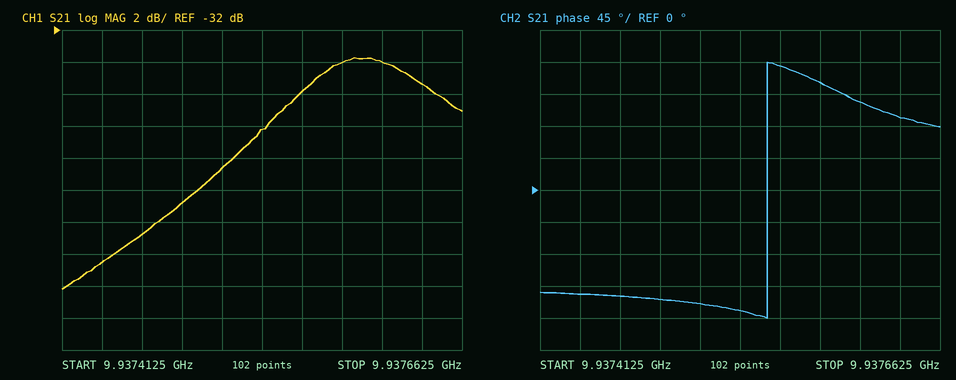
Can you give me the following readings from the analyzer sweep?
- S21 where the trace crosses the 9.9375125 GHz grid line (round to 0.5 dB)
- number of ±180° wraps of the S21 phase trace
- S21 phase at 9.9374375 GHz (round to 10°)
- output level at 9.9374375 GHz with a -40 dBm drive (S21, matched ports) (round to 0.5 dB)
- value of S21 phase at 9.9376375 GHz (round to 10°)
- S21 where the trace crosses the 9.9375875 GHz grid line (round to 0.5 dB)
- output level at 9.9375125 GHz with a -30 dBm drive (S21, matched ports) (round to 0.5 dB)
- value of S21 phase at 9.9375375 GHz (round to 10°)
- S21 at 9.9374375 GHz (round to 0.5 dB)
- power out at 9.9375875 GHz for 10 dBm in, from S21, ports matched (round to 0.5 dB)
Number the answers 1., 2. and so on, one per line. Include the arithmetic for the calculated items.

1. -40.5 dB
2. 1
3. -150°
4. -40 dBm + (-46.5 dB) = -86.5 dBm
5. 100°
6. -34.0 dB
7. -30 dBm + (-40.5 dB) = -70.5 dBm
8. -170°
9. -46.5 dB
10. 10 dBm + (-34.0 dB) = -24.0 dBm
